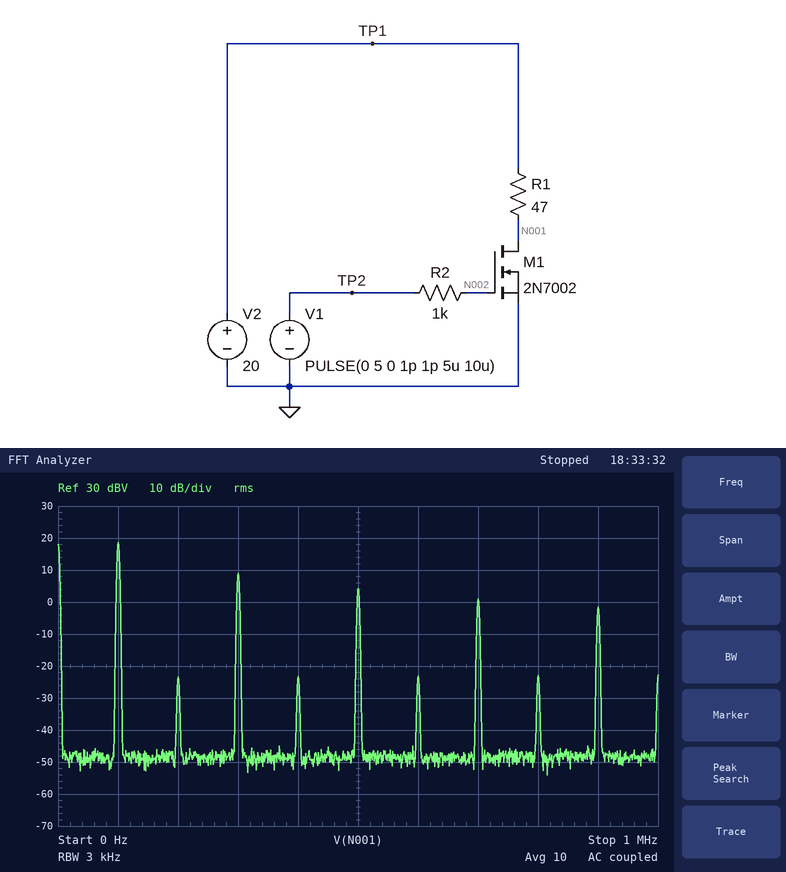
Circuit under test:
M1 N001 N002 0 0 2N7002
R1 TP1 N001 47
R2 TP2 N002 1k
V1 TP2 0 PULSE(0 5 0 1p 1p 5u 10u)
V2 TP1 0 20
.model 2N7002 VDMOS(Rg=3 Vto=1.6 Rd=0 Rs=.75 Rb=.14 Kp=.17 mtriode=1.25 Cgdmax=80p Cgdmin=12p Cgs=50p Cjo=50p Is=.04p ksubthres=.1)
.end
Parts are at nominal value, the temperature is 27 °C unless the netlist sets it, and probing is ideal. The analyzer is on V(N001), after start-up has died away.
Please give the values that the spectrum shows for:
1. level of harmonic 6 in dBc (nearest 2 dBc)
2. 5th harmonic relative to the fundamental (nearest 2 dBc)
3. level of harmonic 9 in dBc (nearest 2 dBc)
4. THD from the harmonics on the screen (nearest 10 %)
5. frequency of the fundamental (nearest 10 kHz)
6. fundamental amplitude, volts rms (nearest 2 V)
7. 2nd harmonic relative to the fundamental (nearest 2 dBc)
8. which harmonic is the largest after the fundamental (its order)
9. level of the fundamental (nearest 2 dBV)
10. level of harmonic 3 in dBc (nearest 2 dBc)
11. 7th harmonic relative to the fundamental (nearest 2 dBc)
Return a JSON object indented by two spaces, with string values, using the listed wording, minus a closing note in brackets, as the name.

{
  "level of harmonic 6 in dBc": "-42 dBc",
  "5th harmonic relative to the fundamental": "-14 dBc",
  "level of harmonic 9 in dBc": "-20 dBc",
  "THD from the harmonics on the screen": "40 %",
  "frequency of the fundamental": "100 kHz",
  "fundamental amplitude, volts rms": "8 V",
  "2nd harmonic relative to the fundamental": "-42 dBc",
  "which harmonic is the largest after the fundamental": "3",
  "level of the fundamental": "18 dBV",
  "level of harmonic 3 in dBc": "-10 dBc",
  "7th harmonic relative to the fundamental": "-18 dBc"
}
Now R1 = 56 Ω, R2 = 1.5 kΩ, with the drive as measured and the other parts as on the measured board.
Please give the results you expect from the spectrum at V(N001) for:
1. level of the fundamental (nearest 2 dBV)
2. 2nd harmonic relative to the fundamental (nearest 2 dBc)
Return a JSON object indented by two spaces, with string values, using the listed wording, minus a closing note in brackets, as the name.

{
  "level of the fundamental": "18 dBV",
  "2nd harmonic relative to the fundamental": "-48 dBc"
}
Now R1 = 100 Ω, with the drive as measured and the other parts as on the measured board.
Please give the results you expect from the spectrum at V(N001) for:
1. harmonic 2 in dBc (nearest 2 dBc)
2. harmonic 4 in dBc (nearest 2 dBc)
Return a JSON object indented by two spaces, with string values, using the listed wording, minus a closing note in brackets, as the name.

{
  "harmonic 2 in dBc": "-34 dBc",
  "harmonic 4 in dBc": "-34 dBc"
}
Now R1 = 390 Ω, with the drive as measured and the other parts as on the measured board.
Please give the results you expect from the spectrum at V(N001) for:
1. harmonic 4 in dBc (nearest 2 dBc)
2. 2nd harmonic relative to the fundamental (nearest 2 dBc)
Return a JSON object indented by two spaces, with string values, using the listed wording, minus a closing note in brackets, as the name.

{
  "harmonic 4 in dBc": "-26 dBc",
  "2nd harmonic relative to the fundamental": "-26 dBc"
}
